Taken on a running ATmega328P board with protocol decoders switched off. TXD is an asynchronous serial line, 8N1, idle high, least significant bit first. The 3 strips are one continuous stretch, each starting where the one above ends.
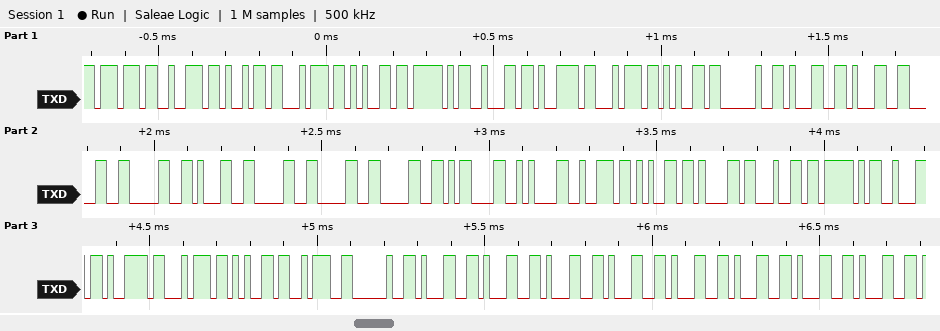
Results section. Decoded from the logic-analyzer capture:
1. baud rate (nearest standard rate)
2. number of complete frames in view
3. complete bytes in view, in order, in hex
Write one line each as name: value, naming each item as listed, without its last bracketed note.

baud rate: 57600 baud
number of complete frames in view: 40
complete bytes in view, in order, in hex: 0x77 0x72 0x69 0x74 0x65 0x5F 0x62 0x79 0x74 0x65 0x20 0x31 0x31 0x30 0x30 0x31 0x30 0x30 0x30 0x0D 0x0A 0x72 0x65 0x61 0x64 0x5F 0x62 0x79 0x74 0x65 0x3A 0x20 0x31 0x31 0x31 0x31 0x31 0x31 0x31 0x31
